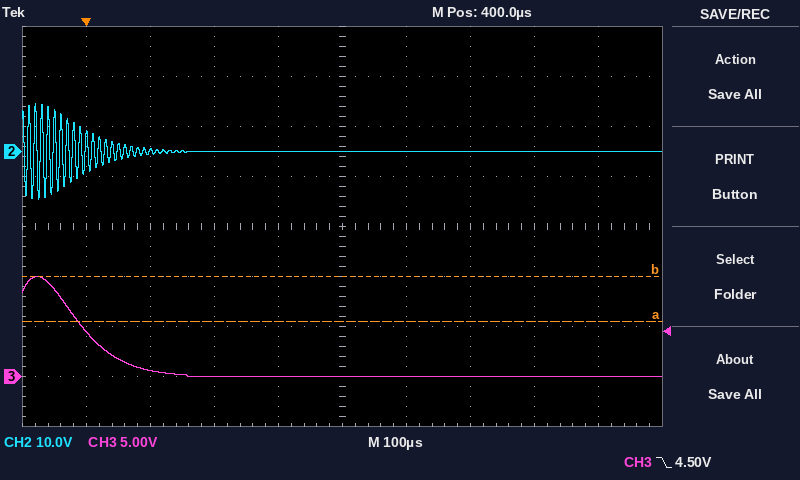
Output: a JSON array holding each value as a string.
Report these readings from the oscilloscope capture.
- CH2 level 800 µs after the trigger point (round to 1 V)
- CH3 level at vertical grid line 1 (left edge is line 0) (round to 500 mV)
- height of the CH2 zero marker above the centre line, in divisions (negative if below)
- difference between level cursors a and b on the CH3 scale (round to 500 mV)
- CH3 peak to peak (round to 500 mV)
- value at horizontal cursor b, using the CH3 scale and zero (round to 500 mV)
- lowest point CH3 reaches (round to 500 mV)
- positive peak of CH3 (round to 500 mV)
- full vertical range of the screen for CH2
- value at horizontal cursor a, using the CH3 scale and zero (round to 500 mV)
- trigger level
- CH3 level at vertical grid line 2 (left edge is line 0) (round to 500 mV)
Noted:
["0 V", "4.5 V", "+1.5 div", "4.5 V", "10.0 V", "10.0 V", "0.0 V", "10.0 V", "80 V", "5.5 V", "4.50 V", "500 mV"]
